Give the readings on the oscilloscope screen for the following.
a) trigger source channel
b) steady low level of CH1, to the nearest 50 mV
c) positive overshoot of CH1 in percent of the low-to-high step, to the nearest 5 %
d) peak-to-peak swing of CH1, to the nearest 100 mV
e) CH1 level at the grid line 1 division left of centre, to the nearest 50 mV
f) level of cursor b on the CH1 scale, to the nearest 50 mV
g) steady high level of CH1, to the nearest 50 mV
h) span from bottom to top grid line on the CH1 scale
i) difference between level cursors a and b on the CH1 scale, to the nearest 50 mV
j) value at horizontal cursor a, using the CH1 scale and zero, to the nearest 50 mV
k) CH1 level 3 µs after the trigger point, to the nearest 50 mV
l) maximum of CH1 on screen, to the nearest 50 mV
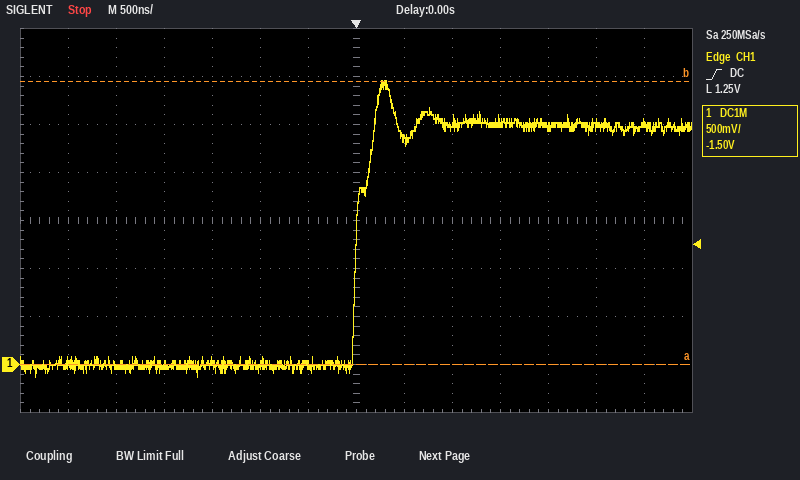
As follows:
CH1
0 mV
20 %
3.10 V
0 mV
2.95 V
2.50 V
4 V
2.95 V
0 mV
2.50 V
2.95 V
